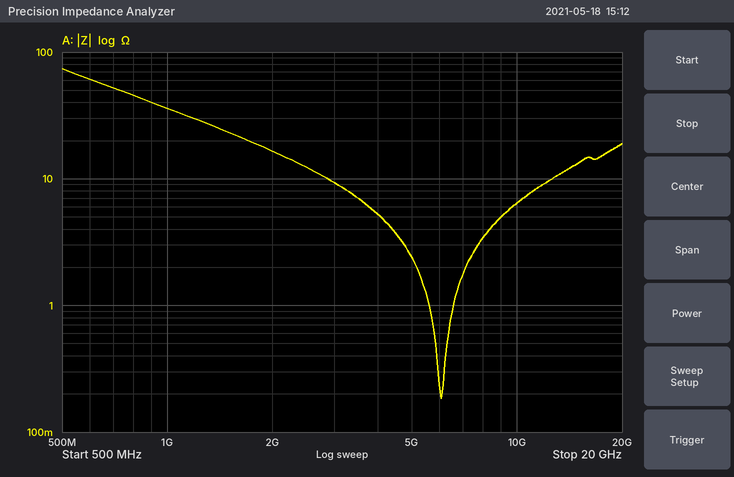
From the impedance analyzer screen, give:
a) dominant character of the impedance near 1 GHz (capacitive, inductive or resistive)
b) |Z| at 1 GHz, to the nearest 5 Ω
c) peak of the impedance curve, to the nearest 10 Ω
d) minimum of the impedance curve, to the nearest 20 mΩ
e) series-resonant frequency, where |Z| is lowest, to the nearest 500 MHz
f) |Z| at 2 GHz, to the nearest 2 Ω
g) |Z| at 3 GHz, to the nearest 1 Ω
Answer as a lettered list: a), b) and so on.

a) capacitive
b) 35 Ω
c) 70 Ω
d) 180 mΩ
e) 6.0 GHz
f) 16 Ω
g) 9 Ω
